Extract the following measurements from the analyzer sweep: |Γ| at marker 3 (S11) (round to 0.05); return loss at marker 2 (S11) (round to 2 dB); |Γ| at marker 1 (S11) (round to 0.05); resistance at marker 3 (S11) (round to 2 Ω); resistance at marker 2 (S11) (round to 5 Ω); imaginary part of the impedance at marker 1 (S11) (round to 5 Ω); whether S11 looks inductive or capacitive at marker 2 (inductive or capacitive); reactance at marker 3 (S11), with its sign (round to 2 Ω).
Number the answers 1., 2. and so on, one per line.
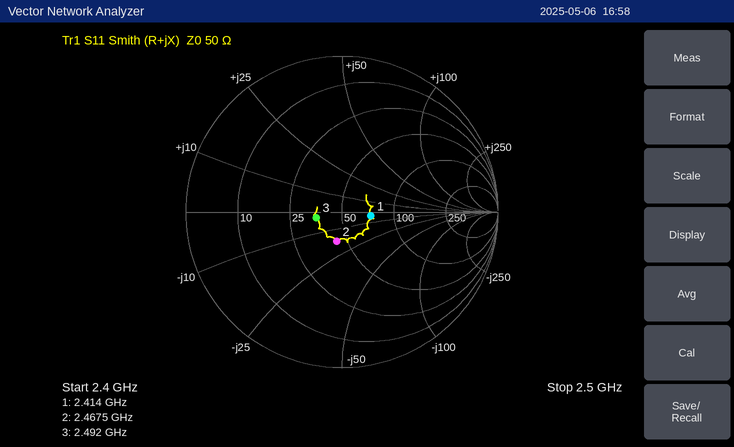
1. 0.15
2. 14 dB
3. 0.20
4. 36 Ω
5. 45 Ω
6. -5 Ω
7. capacitive
8. -2 Ω
